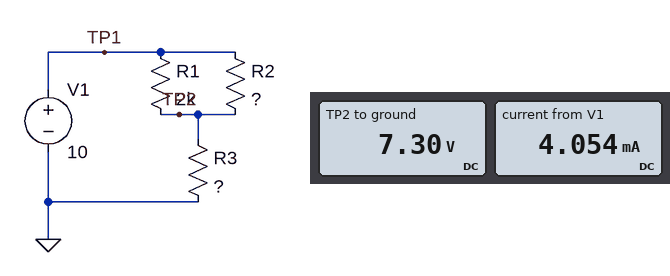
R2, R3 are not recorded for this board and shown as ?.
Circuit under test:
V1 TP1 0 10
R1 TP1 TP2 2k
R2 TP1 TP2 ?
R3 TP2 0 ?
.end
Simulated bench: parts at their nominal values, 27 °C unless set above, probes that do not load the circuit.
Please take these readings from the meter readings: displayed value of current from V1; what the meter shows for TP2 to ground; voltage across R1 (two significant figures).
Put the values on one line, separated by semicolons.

4.054 mA; 7.30 V; 2.7 V
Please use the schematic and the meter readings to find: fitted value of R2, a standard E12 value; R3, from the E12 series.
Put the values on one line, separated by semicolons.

1 kΩ; 1.8 kΩ
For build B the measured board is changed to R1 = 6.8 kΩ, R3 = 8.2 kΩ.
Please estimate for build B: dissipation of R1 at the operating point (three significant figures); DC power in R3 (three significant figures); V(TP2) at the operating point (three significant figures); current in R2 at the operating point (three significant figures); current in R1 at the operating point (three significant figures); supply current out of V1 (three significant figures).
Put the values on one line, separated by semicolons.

136 µW; 9.96 mW; 9.04 V; 961 µA; 141 µA; 1.10 mA
